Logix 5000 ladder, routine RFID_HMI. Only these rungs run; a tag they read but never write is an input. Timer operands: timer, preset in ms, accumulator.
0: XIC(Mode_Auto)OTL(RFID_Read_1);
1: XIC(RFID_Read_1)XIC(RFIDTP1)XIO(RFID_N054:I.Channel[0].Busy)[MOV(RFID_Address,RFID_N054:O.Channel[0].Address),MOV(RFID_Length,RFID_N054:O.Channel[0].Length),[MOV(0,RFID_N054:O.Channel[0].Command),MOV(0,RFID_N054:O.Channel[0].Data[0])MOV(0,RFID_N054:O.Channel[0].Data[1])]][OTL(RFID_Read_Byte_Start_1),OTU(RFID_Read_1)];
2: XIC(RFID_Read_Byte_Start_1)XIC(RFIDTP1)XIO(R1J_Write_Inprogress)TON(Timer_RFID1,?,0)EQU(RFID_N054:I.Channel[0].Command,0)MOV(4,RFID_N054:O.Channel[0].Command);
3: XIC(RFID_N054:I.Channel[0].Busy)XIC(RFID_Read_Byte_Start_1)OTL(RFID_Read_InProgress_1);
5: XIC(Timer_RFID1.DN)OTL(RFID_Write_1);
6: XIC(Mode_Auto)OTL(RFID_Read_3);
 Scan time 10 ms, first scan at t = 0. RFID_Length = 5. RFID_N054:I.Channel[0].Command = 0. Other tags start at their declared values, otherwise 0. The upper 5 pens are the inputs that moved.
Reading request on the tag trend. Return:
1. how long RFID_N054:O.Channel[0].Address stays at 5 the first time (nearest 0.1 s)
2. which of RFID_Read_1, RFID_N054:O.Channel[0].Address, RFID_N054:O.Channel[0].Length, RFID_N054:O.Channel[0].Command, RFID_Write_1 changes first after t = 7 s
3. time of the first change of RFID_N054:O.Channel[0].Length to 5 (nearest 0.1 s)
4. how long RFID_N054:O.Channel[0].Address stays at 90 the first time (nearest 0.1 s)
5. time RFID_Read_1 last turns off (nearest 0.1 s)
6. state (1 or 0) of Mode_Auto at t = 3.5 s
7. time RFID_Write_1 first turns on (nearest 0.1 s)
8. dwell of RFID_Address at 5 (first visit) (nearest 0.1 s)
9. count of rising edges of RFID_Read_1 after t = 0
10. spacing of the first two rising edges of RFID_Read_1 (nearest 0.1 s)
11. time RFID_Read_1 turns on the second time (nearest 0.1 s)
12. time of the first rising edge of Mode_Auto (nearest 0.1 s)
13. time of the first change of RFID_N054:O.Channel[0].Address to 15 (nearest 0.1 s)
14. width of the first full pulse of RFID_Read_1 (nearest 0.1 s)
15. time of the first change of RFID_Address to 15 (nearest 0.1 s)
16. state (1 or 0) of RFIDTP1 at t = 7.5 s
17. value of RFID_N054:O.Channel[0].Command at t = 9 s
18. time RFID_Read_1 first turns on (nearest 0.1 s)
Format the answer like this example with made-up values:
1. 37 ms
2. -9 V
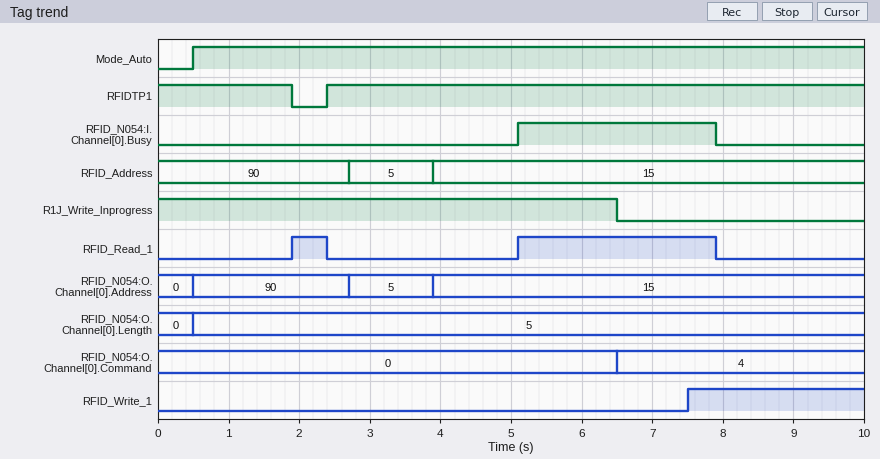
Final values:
1. 1.2 s
2. RFID_Write_1
3. 0.5 s
4. 2.2 s
5. 7.9 s
6. 1
7. 7.5 s
8. 1.2 s
9. 2
10. 3.2 s
11. 5.1 s
12. 0.5 s
13. 3.9 s
14. 0.5 s
15. 3.9 s
16. 1
17. 4
18. 1.9 s
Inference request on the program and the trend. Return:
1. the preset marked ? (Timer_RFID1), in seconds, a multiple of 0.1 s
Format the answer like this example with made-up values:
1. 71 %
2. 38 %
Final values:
1. 1.0 s
